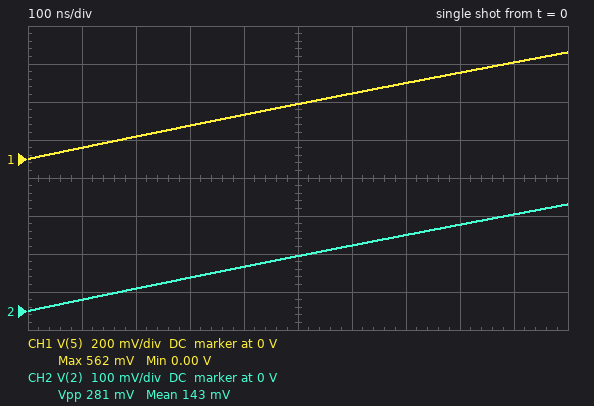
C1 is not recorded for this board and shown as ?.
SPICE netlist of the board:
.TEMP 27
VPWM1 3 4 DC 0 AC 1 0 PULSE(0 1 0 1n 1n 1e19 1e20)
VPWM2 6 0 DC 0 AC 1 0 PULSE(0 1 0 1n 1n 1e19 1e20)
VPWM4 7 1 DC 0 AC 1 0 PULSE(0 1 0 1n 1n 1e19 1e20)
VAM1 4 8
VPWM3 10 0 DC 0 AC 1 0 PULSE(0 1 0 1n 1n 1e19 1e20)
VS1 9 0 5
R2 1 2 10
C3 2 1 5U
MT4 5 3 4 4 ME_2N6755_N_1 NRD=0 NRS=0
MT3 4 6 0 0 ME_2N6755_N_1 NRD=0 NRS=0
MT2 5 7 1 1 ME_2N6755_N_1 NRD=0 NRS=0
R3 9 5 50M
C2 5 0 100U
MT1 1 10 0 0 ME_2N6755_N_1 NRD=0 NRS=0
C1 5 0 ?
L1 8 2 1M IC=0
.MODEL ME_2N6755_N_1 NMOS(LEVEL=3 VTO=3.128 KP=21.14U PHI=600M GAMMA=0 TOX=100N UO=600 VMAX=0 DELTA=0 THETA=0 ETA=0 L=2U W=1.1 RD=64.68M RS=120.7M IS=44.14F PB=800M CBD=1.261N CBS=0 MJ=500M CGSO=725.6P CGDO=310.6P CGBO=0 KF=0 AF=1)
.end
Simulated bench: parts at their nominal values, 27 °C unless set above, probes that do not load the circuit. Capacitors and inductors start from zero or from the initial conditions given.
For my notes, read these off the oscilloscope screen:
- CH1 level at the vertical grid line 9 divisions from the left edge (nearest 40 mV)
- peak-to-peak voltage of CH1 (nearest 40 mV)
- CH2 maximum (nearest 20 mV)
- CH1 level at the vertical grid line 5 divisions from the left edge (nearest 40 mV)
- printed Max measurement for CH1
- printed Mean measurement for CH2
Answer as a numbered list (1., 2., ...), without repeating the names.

1. 520 mV
2. 560 mV
3. 280 mV
4. 280 mV
5. 562 mV
6. 143 mV
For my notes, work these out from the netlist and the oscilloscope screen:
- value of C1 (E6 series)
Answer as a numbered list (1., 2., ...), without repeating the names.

1. 68 µF
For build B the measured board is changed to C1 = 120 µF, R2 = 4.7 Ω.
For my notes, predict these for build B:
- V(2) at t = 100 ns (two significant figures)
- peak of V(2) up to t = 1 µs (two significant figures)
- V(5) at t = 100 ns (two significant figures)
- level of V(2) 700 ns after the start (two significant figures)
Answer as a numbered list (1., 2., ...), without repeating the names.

1. 23 mV
2. 220 mV
3. 45 mV
4. 150 mV
